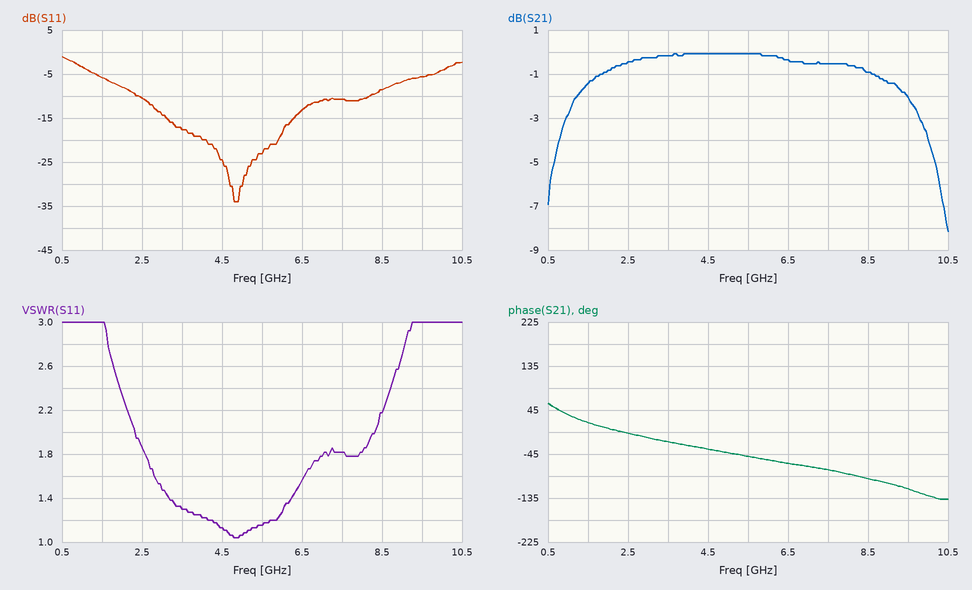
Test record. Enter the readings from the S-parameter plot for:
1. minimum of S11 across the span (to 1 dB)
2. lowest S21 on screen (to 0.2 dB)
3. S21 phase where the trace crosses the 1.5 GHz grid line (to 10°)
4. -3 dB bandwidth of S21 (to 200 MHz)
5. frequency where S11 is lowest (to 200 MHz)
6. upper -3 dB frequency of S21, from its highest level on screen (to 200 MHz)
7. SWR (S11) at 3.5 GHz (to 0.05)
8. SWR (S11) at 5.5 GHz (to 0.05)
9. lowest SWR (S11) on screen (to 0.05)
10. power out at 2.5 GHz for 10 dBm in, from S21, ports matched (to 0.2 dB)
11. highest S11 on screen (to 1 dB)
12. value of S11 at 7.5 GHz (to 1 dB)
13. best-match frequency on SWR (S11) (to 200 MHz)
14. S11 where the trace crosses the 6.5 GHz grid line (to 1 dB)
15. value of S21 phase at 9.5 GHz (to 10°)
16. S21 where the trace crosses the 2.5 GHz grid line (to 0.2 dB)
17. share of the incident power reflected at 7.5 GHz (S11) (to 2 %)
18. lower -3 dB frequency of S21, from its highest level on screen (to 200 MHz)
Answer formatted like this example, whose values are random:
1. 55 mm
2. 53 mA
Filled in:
1. -34 dB
2. -8.2 dB
3. 20°
4. 8.8 GHz
5. 4.8 GHz
6. 9.8 GHz
7. 1.30
8. 1.15
9. 1.05
10. 9.6 dBm
11. -1 dB
12. -11 dB
13. 4.8 GHz
14. -13 dB
15. -120°
16. -0.4 dB
17. 8 %
18. 1.0 GHz
